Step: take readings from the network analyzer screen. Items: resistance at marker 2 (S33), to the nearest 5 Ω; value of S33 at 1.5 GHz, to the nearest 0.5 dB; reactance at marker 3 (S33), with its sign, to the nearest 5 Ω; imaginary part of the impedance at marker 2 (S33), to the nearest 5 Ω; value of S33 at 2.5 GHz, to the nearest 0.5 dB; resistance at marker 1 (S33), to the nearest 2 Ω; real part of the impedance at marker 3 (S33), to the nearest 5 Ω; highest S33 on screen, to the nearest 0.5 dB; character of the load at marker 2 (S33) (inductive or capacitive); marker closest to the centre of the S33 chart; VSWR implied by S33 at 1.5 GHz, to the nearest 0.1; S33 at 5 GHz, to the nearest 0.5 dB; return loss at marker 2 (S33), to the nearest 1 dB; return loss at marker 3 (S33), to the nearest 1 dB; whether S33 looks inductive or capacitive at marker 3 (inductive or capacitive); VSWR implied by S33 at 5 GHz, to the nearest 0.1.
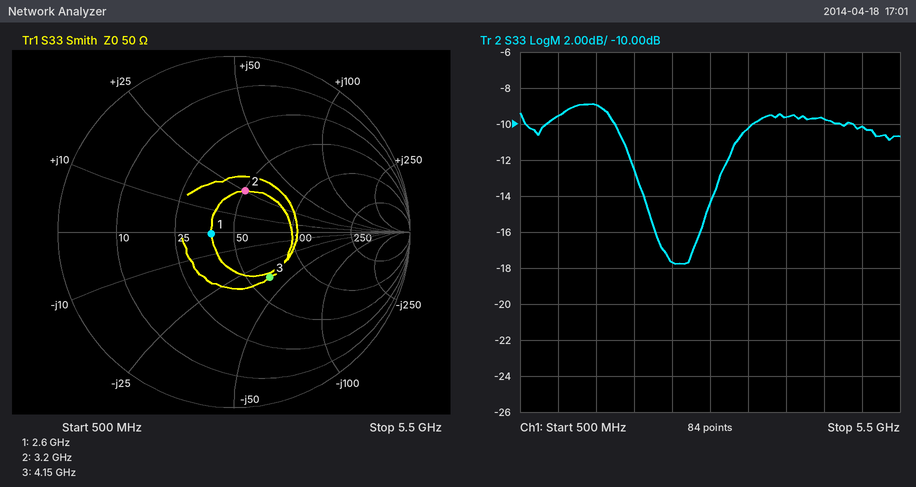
50 Ω
-9.0 dB
-35 Ω
+25 Ω
-17.5 dB
38 Ω
65 Ω
-9.0 dB
inductive
marker 1
2.1
-10.0 dB
12 dB
10 dB
capacitive
1.9
